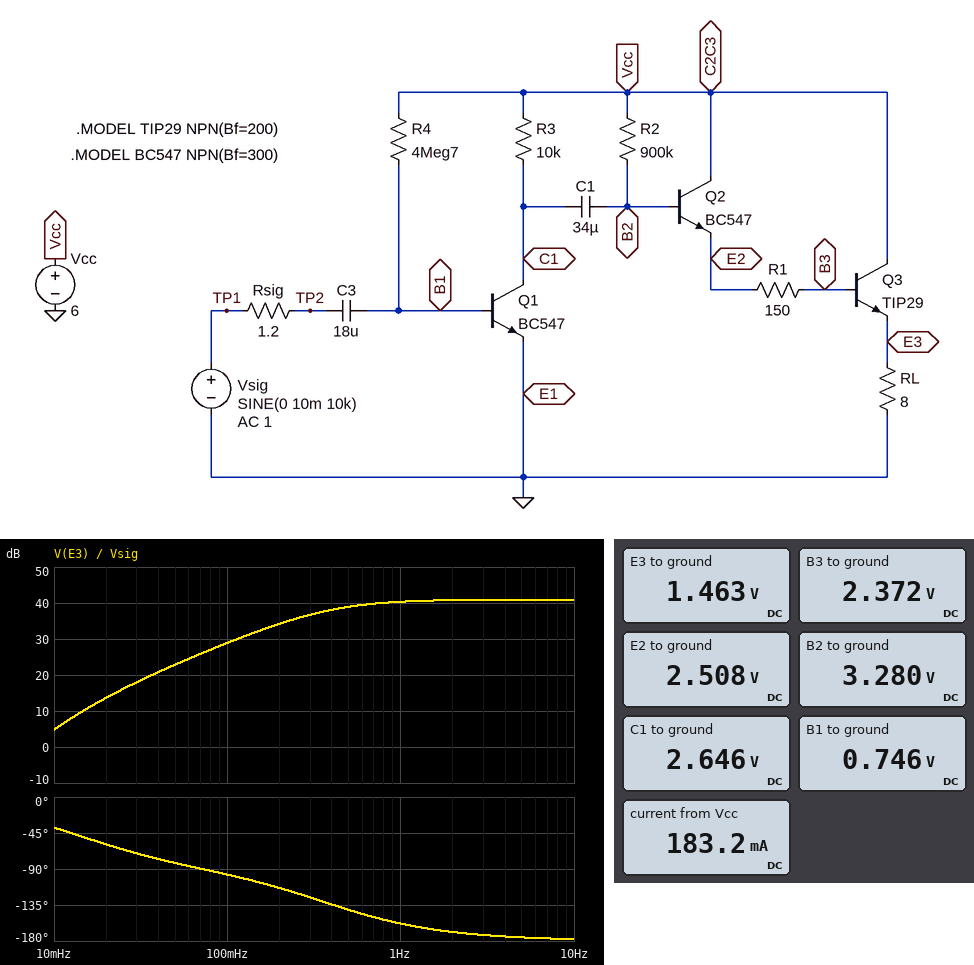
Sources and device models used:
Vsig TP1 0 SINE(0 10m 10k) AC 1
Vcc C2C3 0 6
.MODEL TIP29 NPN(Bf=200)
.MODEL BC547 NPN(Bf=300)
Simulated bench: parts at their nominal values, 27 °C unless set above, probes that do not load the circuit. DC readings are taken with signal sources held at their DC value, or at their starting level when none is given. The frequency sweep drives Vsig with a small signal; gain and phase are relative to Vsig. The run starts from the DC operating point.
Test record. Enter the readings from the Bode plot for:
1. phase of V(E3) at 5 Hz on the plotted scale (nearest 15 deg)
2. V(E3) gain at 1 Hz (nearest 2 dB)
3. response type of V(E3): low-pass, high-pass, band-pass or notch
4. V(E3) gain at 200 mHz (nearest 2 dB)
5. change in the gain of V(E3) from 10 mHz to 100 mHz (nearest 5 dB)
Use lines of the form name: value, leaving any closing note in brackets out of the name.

phase of V(E3) at 5 Hz on the plotted scale: -180 deg
V(E3) gain at 1 Hz: 40 dB
response type of V(E3): low-pass, high-pass, band-pass or notch: high-pass
V(E3) gain at 200 mHz: 34 dB
change in the gain of V(E3) from 10 mHz to 100 mHz: 25 dB
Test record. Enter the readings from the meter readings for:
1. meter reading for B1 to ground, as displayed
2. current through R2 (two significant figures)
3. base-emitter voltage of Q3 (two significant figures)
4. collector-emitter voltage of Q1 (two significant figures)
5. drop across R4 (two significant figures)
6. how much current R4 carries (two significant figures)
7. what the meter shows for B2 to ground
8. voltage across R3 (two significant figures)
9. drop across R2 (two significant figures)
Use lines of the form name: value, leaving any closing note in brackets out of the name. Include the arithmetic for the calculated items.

meter reading for B1 to ground, as displayed: 0.746 V
current through R2: (6 V - 3.28 V) / 900 kΩ = 3.0 µA
base-emitter voltage of Q3: 2.372 V - 1.463 V = 910 mV
collector-emitter voltage of Q1: 2.646 V = 2.6 V
drop across R4: 6 V - 746 mV = 5.3 V
how much current R4 carries: (6 V - 746 mV) / 4.7 MΩ = 1.1 µA
what the meter shows for B2 to ground: 3.280 V
voltage across R3: 6 V - 2.646 V = 3.4 V
drop across R2: 6 V - 3.28 V = 2.7 V
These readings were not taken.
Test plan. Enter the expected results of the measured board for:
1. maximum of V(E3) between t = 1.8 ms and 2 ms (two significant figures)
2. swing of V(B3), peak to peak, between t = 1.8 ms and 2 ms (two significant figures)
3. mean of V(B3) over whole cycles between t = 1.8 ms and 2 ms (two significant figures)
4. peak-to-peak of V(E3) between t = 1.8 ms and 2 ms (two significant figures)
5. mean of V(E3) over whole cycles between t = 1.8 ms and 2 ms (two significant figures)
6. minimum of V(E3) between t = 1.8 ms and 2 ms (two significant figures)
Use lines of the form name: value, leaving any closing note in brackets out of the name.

maximum of V(E3) between t = 1.8 ms and 2 ms: 2.4 V
swing of V(B3), peak to peak, between t = 1.8 ms and 2 ms: 2.3 V
mean of V(B3) over whole cycles between t = 1.8 ms and 2 ms: 2.3 V
peak-to-peak of V(E3) between t = 1.8 ms and 2 ms: 2.2 V
mean of V(E3) over whole cycles between t = 1.8 ms and 2 ms: 1.4 V
minimum of V(E3) between t = 1.8 ms and 2 ms: 160 mV
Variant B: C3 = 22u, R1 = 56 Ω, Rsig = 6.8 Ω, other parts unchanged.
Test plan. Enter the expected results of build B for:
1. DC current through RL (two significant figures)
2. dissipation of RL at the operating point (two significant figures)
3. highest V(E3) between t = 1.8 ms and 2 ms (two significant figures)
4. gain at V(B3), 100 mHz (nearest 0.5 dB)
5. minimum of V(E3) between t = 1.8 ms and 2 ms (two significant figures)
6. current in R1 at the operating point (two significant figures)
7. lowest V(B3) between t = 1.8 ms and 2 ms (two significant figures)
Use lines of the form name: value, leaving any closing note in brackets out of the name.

DC current through RL: 190 mA
dissipation of RL at the operating point: 280 mW
highest V(E3) between t = 1.8 ms and 2 ms: 2.5 V
gain at V(B3), 100 mHz: 31.0 dB
minimum of V(E3) between t = 1.8 ms and 2 ms: 130 mV
current in R1 at the operating point: 930 µA
lowest V(B3) between t = 1.8 ms and 2 ms: 980 mV
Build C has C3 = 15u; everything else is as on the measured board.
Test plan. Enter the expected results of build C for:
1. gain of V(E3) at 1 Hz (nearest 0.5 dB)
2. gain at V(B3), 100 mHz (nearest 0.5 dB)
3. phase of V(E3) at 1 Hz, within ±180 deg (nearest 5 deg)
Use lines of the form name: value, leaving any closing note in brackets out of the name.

gain of V(E3) at 1 Hz: 40.0 dB
gain at V(B3), 100 mHz: 27.5 dB
phase of V(E3) at 1 Hz, within ±180 deg: -155 deg
